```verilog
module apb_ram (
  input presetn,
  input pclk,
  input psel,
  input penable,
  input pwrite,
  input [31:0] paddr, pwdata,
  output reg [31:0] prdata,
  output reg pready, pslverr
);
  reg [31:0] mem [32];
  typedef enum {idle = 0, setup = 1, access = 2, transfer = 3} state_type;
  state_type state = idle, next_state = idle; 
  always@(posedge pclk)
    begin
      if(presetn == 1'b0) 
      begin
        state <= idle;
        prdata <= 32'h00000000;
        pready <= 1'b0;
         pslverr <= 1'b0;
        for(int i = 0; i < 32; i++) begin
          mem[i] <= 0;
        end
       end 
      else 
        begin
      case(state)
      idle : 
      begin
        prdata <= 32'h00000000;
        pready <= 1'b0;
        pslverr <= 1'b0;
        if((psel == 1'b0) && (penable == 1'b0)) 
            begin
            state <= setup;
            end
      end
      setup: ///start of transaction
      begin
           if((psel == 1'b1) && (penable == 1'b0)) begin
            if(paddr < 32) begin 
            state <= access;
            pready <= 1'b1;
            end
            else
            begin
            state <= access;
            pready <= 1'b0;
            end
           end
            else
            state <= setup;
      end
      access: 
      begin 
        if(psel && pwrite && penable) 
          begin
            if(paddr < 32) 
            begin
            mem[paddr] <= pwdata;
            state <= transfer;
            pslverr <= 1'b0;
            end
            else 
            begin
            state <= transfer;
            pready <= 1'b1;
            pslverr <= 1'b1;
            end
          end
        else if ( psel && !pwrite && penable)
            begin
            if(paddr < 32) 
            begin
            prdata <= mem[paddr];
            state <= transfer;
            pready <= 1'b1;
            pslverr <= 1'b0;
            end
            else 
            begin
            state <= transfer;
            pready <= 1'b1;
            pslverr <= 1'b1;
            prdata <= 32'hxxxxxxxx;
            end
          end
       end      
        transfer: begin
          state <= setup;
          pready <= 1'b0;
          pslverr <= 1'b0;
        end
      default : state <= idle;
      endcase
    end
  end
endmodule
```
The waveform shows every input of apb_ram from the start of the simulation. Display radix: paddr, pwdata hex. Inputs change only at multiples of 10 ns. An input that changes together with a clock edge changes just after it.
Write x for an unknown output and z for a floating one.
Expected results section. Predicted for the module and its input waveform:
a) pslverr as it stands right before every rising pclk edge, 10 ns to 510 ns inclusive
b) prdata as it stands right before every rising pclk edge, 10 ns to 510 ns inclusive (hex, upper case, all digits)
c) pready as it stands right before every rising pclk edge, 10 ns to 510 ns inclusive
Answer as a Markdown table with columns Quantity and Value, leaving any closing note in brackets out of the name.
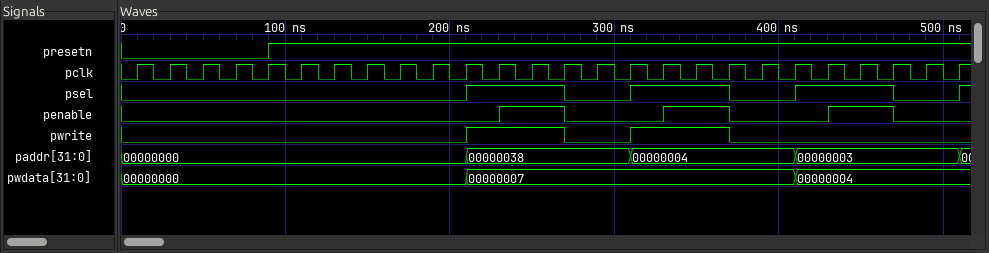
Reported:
| Quantity | Value |
|---|---|
| pslverr as it stands right before every rising pclk edge, 10 ns to 510 ns inclusive | x 0 0 0 0 0 0 0 0 0 0 0 0 1 0 0 0 0 0 0 0 0 0 0 0 0 |
| prdata as it stands right before every rising pclk edge, 10 ns to 510 ns inclusive | x, 00000000, 00000000, 00000000, 00000000, 00000000, 00000000, 00000000, 00000000, 00000000, 00000000, 00000000, 00000000, 00000000, 00000000, 00000000, 00000000, 00000000, 00000000, 00000000, 00000000, 00000000, 00000000, 00000000, 00000000, 00000000 |
| pready as it stands right before every rising pclk edge, 10 ns to 510 ns inclusive | x 0 0 0 0 0 0 0 0 0 0 0 0 1 0 0 0 1 1 0 0 0 1 1 0 0 |
